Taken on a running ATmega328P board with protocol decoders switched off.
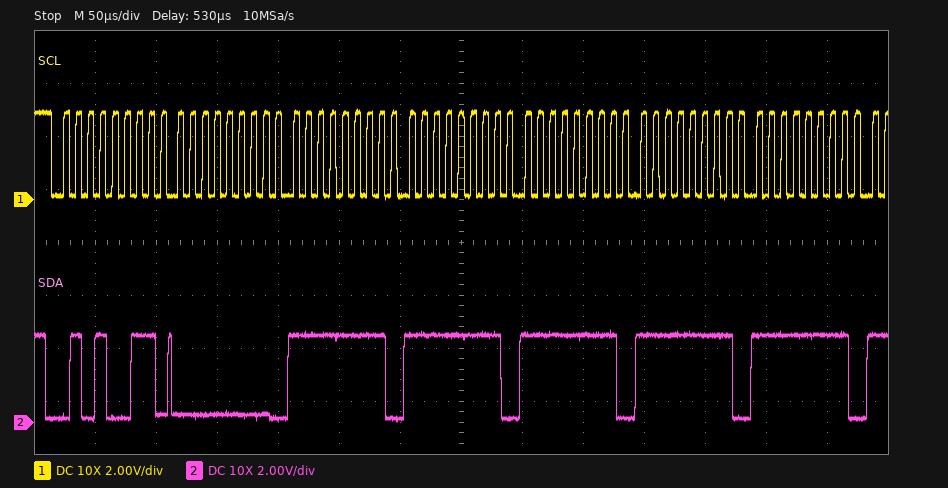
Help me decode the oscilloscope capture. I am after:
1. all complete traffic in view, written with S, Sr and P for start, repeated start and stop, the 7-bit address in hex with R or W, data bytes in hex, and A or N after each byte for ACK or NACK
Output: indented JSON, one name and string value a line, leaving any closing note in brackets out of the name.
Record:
{
  "all complete traffic in view, written with S, Sr and P for start, repeated start and stop, the 7-bit address in hex with R or W, data bytes in hex, and A or N after each byte for ACK or NACK": "S 29R A 00 A FF A FF A FF A FF A FF A"
}
